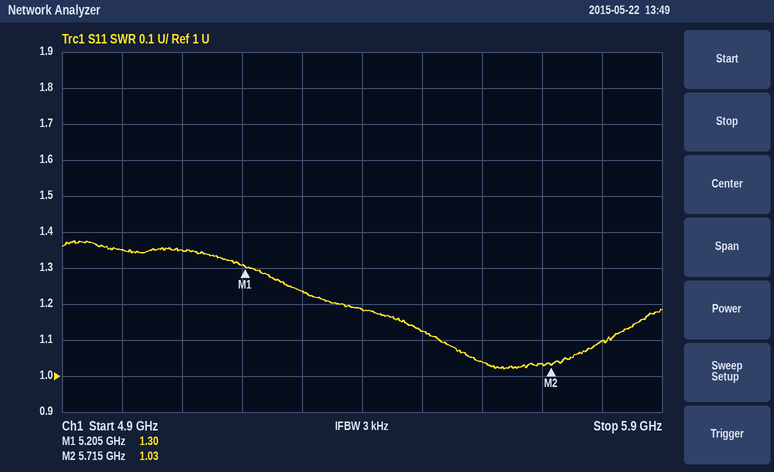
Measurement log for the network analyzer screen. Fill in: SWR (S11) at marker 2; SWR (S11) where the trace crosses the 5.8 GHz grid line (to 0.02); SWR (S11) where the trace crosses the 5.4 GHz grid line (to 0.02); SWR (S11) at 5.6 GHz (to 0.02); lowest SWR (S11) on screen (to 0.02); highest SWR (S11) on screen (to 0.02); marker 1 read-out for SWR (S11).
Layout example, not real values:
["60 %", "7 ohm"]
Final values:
["1.03", "1.10", "1.18", "1.04", "1.02", "1.38", "1.30"]
